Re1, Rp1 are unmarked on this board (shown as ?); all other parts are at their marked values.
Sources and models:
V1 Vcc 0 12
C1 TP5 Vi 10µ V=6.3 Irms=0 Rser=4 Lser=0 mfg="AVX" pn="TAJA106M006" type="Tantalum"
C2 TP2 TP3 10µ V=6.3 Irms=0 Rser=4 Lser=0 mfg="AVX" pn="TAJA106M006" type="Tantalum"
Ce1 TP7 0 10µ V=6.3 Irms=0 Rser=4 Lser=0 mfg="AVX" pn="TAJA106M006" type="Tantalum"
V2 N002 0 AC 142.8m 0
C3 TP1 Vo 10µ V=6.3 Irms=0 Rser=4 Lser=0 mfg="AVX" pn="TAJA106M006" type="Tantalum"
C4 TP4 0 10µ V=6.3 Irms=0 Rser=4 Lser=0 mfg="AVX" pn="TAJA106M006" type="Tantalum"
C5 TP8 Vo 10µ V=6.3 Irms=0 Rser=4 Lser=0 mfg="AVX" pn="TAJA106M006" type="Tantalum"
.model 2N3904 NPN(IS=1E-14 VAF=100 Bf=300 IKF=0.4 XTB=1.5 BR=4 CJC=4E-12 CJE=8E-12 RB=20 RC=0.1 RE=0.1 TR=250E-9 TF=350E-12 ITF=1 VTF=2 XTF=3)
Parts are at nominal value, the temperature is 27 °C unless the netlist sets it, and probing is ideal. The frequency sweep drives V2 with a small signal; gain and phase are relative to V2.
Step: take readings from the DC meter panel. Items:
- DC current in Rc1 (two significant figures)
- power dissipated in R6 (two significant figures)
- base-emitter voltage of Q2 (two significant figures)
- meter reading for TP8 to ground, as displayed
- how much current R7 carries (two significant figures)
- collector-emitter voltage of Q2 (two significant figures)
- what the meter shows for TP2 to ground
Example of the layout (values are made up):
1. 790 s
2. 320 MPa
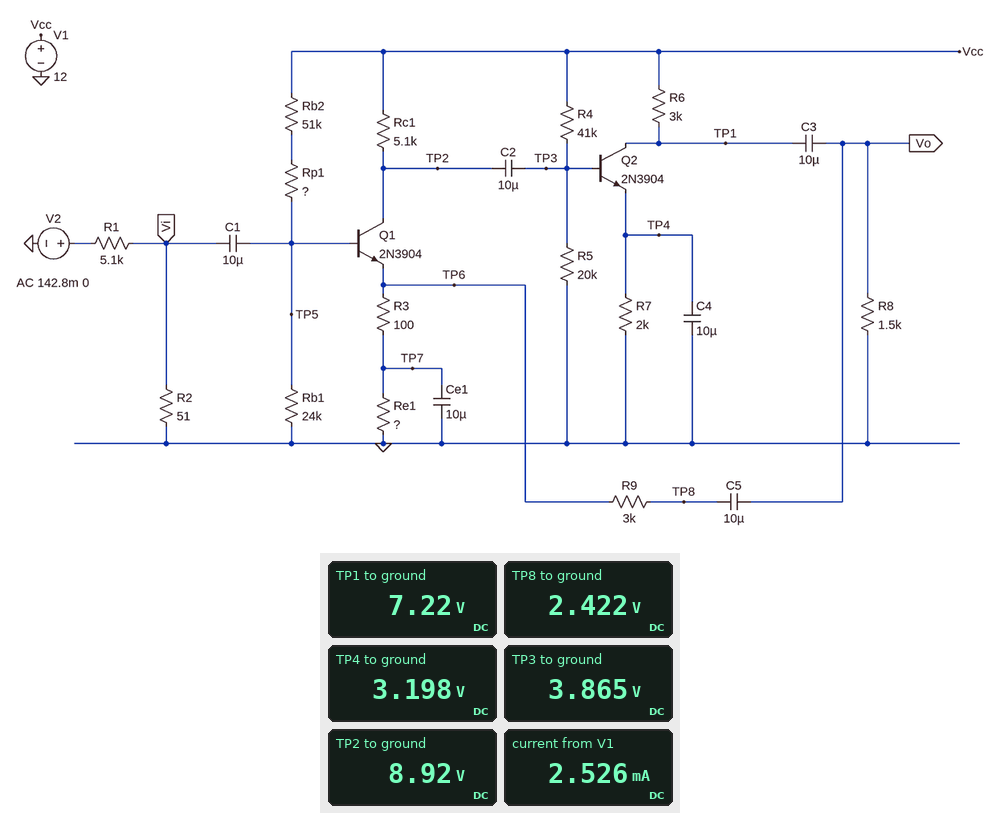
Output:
1. 600 µA
2. 7.6 mW
3. 670 mV
4. 2.422 V
5. 1.6 mA
6. 4.0 V
7. 8.92 V
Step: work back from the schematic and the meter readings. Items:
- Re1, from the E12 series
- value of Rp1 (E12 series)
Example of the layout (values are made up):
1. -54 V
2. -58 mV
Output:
1. 3.9 kΩ
2. 18 kΩ
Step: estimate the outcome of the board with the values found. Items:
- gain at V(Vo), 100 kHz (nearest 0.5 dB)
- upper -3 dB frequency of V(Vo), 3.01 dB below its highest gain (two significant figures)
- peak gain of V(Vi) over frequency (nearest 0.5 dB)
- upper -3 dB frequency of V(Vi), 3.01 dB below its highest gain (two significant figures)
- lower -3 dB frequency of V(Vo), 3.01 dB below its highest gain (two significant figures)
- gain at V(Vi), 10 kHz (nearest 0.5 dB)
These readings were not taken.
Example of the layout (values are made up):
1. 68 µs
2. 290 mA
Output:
1. -11.0 dB
2. 14 MHz
3. -40.0 dB
4. 320 MHz
5. 160 Hz
6. -40.0 dB
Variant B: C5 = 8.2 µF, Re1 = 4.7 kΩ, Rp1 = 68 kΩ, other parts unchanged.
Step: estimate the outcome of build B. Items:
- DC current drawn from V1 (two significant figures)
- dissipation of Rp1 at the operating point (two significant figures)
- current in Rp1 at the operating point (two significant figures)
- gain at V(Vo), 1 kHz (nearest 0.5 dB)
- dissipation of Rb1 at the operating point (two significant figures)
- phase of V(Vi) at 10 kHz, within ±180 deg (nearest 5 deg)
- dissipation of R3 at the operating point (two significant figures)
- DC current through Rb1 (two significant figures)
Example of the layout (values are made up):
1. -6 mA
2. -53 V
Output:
1. 2.2 mA
2. 480 µW
3. 84 µA
4. -11.5 dB
5. 170 µW
6. 0 deg
7. 8.2 µW
8. 83 µA
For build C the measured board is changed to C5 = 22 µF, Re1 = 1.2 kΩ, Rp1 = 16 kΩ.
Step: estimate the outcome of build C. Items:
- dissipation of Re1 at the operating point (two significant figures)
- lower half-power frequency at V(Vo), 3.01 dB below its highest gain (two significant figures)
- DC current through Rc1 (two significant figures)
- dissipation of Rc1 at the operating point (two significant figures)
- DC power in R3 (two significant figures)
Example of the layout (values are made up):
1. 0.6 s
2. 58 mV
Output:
1. 4.0 mW
2. 170 Hz
3. 1.8 mA
4. 17 mW
5. 340 µW
